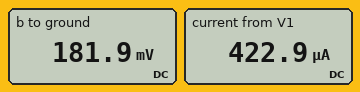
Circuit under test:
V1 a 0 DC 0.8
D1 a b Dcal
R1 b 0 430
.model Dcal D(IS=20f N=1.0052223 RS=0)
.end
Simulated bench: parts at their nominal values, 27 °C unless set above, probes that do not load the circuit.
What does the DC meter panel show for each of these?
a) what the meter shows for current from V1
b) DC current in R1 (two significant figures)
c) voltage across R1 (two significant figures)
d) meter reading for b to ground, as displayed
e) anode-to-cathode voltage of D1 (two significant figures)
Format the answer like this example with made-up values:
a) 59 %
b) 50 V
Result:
a) 422.9 µA
b) 420 µA
c) 180 mV
d) 181.9 mV
e) 620 mV
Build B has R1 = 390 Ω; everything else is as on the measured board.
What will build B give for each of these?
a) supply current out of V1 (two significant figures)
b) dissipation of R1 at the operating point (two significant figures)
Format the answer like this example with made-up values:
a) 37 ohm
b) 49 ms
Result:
a) 460 µA
b) 83 µW
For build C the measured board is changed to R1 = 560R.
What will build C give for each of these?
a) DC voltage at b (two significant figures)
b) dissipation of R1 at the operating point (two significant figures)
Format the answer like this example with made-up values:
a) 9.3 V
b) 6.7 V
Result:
a) 190 mV
b) 63 µW
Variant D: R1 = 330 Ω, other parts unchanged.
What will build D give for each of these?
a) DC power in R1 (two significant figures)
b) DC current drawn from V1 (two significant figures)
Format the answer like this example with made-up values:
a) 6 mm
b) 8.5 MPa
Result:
a) 94 µW
b) 530 µA
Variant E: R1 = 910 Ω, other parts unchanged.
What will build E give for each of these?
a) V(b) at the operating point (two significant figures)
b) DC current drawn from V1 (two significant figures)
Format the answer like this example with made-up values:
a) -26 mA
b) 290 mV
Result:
a) 200 mV
b) 220 µA
